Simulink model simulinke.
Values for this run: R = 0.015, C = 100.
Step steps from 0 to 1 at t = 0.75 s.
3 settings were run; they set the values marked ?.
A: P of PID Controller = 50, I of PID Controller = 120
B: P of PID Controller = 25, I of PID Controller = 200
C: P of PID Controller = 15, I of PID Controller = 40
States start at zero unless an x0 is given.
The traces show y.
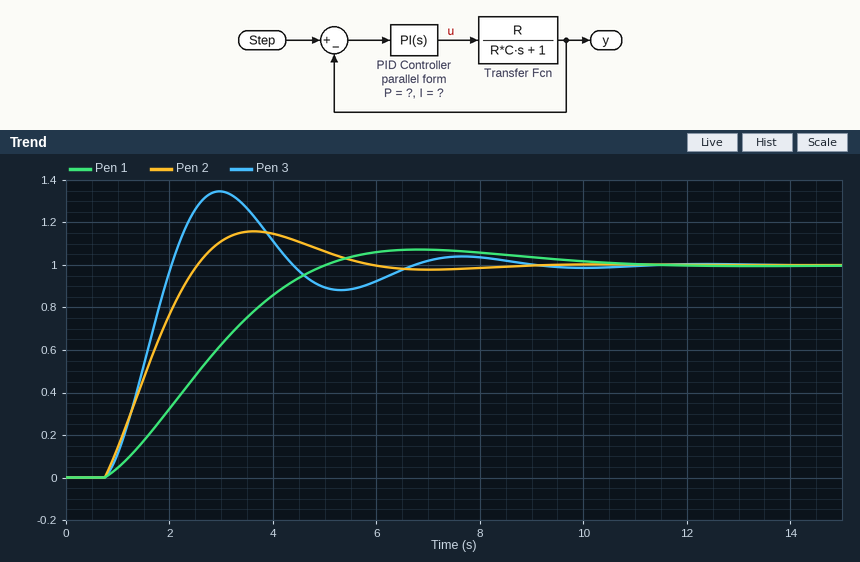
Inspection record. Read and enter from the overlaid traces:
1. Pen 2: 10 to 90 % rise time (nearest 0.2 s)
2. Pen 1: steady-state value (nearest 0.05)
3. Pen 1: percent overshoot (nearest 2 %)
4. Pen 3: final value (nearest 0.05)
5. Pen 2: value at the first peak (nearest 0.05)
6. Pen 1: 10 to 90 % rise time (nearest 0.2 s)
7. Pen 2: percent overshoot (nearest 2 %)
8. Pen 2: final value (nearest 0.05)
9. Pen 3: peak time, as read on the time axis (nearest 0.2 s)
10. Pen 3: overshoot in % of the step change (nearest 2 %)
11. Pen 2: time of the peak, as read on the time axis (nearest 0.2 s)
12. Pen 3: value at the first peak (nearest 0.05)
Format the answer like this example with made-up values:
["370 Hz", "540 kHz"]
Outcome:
["1.4 s", "1.00", "8 %", "1.00", "1.15", "3.0 s", "16 %", "1.00", "3.0 s", "34 %", "3.6 s", "1.35"]
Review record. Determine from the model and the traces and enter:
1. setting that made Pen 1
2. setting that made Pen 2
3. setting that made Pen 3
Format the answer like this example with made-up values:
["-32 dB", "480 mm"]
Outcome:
["C", "A", "B"]
